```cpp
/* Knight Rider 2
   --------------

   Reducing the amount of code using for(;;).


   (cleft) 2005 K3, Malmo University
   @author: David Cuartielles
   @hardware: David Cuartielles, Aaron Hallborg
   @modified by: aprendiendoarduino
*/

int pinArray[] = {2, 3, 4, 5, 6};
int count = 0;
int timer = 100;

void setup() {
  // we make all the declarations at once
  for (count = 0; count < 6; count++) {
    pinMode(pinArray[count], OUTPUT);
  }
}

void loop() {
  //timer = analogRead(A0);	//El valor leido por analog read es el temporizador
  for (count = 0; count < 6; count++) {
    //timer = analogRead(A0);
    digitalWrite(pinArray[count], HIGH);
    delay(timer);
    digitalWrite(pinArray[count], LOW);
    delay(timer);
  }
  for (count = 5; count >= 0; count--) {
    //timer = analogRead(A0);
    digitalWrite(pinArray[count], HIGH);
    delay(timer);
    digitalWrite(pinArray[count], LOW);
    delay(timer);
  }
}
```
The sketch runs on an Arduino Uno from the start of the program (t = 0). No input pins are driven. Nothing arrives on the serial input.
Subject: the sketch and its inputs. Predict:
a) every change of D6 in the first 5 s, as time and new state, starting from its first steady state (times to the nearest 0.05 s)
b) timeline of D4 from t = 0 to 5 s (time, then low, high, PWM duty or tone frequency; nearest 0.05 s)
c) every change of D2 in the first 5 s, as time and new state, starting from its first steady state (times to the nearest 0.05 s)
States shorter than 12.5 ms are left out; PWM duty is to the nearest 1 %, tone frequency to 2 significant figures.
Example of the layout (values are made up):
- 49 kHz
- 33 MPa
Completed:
- 0 s low; 0.8 s high; 0.9 s low; 1.4 s high; 1.5 s low; 3.2 s high; 3.3 s low; 3.8 s high; 3.9 s low
- 0 s low; 0.4 s high; 0.5 s low; 1.8 s high; 1.9 s low; 2.8 s high; 2.9 s low; 4.2 s high; 4.3 s low
- 0 s high; 0.1 s low; 2.2 s high; 2.3 s low; 2.4 s high; 2.5 s low; 4.6 s high; 4.7 s low; 4.8 s high; 4.9 s low
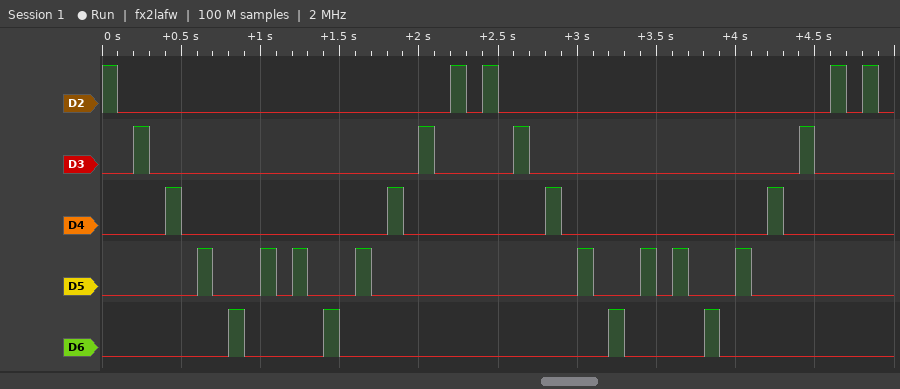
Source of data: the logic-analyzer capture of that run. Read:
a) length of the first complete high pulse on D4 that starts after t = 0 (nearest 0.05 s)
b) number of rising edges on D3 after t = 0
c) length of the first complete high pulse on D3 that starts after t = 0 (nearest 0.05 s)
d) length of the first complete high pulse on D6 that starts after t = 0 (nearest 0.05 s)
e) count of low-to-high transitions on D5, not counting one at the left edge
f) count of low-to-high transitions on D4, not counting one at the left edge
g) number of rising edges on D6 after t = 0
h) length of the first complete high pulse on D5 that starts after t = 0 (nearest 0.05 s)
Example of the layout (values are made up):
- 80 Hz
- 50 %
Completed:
- 0.10 s
- 4
- 0.10 s
- 0.10 s
- 8
- 4
- 4
- 0.10 s
